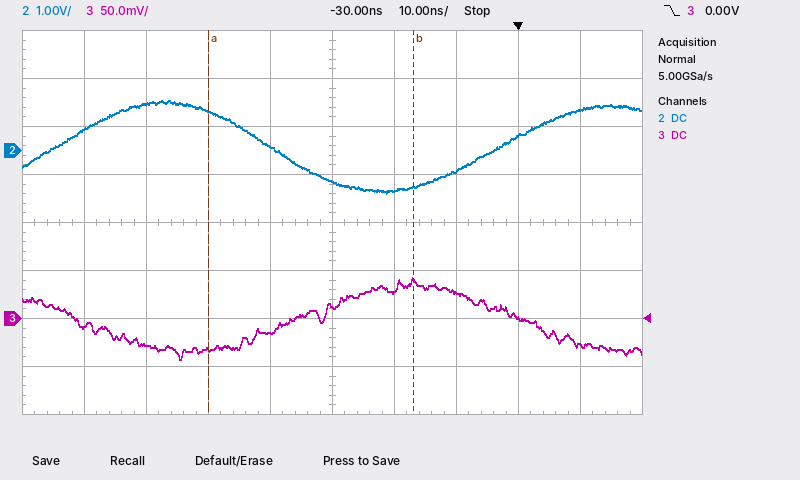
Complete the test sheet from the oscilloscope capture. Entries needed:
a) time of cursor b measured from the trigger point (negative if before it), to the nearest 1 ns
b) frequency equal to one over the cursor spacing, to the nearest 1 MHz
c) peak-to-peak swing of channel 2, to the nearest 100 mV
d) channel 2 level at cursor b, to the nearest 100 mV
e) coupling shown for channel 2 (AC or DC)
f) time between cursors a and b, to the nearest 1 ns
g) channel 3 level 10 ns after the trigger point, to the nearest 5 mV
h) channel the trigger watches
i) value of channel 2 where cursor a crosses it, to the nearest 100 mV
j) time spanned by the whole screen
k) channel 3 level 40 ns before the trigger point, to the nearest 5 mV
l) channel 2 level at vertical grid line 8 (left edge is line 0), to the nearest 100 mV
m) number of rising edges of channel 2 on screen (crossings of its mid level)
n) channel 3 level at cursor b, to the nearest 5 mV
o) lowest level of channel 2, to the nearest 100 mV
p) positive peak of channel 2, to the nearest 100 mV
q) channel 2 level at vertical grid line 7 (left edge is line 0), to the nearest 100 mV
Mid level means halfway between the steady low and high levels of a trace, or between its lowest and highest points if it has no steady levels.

-17 ns
30 MHz
1.9 V
-800 mV
DC
33 ns
-30 mV
channel 3
800 mV
100 ns
-15 mV
300 mV
2
40 mV
-900 mV
1.0 V
-400 mV
